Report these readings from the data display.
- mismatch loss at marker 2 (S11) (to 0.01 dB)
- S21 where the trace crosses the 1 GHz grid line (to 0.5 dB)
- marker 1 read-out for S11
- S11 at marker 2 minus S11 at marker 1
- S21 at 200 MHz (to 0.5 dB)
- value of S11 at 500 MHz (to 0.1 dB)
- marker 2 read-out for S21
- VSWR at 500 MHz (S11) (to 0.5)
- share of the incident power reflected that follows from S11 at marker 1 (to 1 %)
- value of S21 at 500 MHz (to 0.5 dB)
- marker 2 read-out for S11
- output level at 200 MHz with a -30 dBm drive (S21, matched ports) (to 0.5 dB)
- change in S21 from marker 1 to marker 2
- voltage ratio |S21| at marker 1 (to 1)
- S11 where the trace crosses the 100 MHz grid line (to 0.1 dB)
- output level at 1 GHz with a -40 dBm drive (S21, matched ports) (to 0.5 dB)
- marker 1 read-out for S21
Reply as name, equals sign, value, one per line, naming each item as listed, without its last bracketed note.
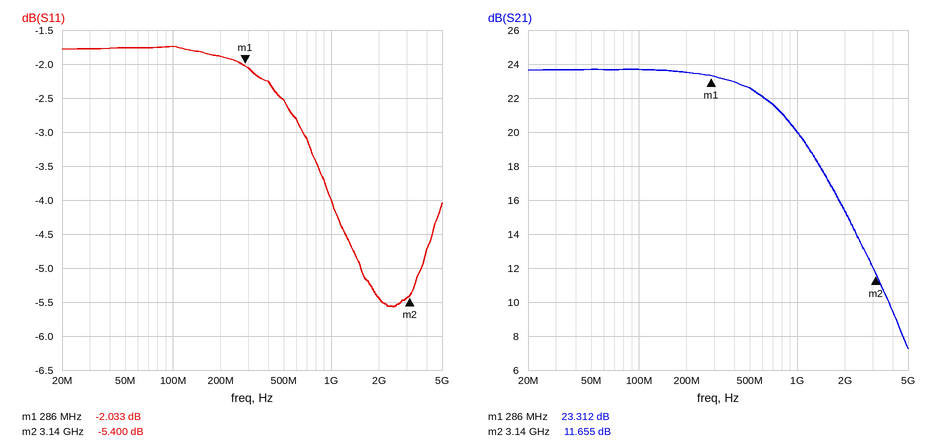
mismatch loss at marker 2 (S11) = 1.48 dB
S21 where the trace crosses the 1 GHz grid line = 20.0 dB
marker 1 read-out for S11 = -2.033 dB
S11 at marker 2 minus S11 at marker 1 = -3.367 dB
S21 at 200 MHz = 23.5 dB
value of S11 at 500 MHz = -2.5 dB
marker 2 read-out for S21 = 11.655 dB
VSWR at 500 MHz (S11) = 7.0
share of the incident power reflected that follows from S11 at marker 1 = 63 %
value of S21 at 500 MHz = 22.5 dB
marker 2 read-out for S11 = -5.400 dB
output level at 200 MHz with a -30 dBm drive (S21, matched ports) = -6.5 dBm
change in S21 from marker 1 to marker 2 = -11.657 dB
voltage ratio |S21| at marker 1 = 15
S11 where the trace crosses the 100 MHz grid line = -1.7 dB
output level at 1 GHz with a -40 dBm drive (S21, matched ports) = -20.0 dBm
marker 1 read-out for S21 = 23.312 dB
